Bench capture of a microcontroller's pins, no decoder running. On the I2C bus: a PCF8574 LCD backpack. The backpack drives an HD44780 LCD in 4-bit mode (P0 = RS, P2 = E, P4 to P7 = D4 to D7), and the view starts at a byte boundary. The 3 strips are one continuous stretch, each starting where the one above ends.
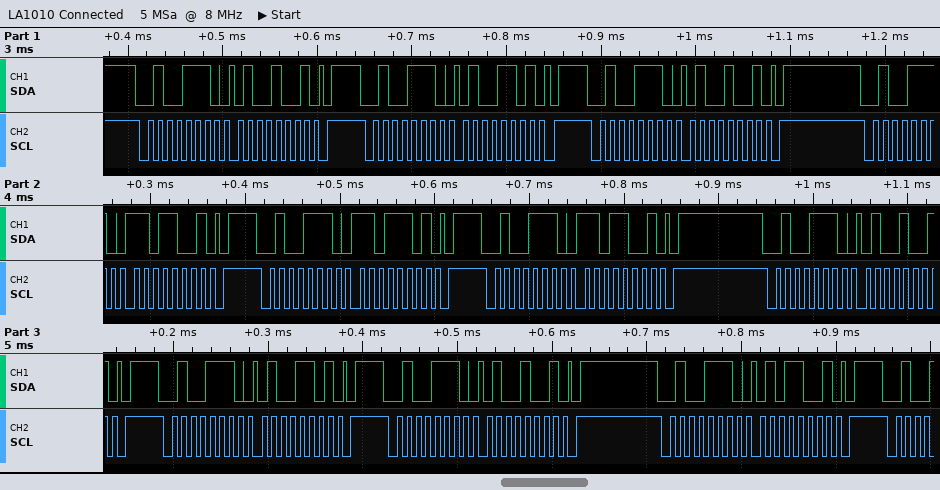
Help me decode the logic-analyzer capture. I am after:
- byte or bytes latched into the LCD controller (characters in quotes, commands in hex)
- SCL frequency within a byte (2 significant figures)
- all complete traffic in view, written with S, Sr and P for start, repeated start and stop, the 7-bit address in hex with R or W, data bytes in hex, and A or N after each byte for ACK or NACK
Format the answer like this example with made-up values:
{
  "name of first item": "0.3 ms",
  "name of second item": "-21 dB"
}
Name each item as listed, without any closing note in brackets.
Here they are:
{
  "byte or bytes latched into the LCD controller": "'M'",
  "SCL frequency within a byte": "100 kHz",
  "all complete traffic in view, written with S, Sr and P for start, repeated start and stop, the 7-bit address in hex with R or W, data bytes in hex, and A or N after each byte for ACK or NACK": "S 27W A 49 A P S 27W A 4D A P S 27W A 49 A P S 27W A D9 A P S 27W A DD A P S 27W A D9 A P S 27W A 49 A P S 27W A 4D A P S 27W A 49 A P S 27W A 59 A P"
}
